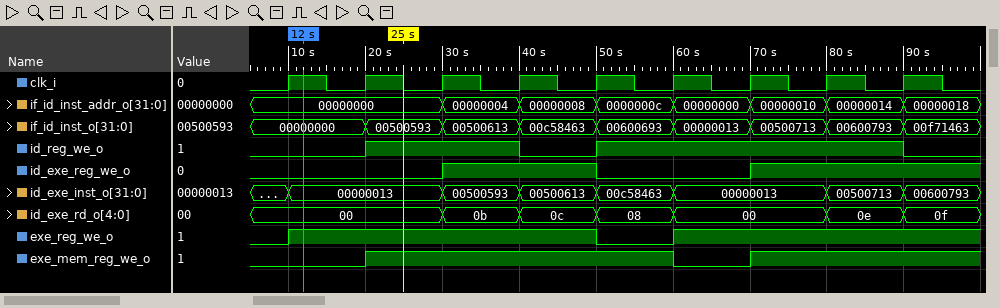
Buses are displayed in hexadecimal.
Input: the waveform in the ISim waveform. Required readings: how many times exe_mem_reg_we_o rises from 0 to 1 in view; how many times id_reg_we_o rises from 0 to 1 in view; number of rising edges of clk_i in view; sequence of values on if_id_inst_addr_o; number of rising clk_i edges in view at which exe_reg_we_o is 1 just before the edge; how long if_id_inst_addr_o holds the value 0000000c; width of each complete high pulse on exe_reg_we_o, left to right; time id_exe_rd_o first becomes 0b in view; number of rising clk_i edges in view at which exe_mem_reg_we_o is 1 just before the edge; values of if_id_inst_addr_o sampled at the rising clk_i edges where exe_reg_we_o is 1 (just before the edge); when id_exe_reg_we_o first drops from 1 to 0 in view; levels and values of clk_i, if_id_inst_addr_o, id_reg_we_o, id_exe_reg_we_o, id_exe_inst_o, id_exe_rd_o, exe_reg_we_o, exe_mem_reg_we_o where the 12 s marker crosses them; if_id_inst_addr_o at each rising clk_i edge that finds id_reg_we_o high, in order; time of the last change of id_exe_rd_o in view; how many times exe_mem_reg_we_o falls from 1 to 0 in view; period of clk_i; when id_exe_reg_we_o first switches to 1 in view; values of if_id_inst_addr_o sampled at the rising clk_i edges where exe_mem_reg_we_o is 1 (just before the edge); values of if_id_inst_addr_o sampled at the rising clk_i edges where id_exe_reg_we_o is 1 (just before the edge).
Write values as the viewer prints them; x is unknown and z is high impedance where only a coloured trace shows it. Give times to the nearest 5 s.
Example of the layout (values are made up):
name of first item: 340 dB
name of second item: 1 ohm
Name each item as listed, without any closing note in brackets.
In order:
how many times exe_mem_reg_we_o rises from 0 to 1 in view: 2
how many times id_reg_we_o rises from 0 to 1 in view: 2
number of rising edges of clk_i in view: 9
sequence of values on if_id_inst_addr_o: 00000000, 00000004, 00000008, 0000000c, 00000000, 00000010, 00000014, 00000018
number of rising clk_i edges in view at which exe_reg_we_o is 1 just before the edge: 7
how long if_id_inst_addr_o holds the value 0000000c: 10 s
width of each complete high pulse on exe_reg_we_o, left to right: 40 s
time id_exe_rd_o first becomes 0b in view: 30 s
number of rising clk_i edges in view at which exe_mem_reg_we_o is 1 just before the edge: 6
values of if_id_inst_addr_o sampled at the rising clk_i edges where exe_reg_we_o is 1: 00000000, 00000000, 00000004, 00000008, 00000000, 00000010, 00000014
when id_exe_reg_we_o first drops from 1 to 0 in view: 50 s
levels and values of clk_i, if_id_inst_addr_o, id_reg_we_o, id_exe_reg_we_o, id_exe_inst_o, id_exe_rd_o, exe_reg_we_o, exe_mem_reg_we_o where the 12 s marker crosses them: clk_i=1, if_id_inst_addr_o=00000000, id_reg_we_o=0, id_exe_reg_we_o=0, id_exe_inst_o=00000013, id_exe_rd_o=00, exe_reg_we_o=1, exe_mem_reg_we_o=0
if_id_inst_addr_o at each rising clk_i edge that finds id_reg_we_o high, in order: 00000000, 00000004, 0000000c, 00000000, 00000010, 00000014
time of the last change of id_exe_rd_o in view: 90 s
how many times exe_mem_reg_we_o falls from 1 to 0 in view: 1
period of clk_i: 10 s
when id_exe_reg_we_o first switches to 1 in view: 30 s
values of if_id_inst_addr_o sampled at the rising clk_i edges where exe_mem_reg_we_o is 1: 00000000, 00000004, 00000008, 0000000c, 00000010, 00000014
values of if_id_inst_addr_o sampled at the rising clk_i edges where id_exe_reg_we_o is 1: 00000004, 00000008, 00000010, 00000014
